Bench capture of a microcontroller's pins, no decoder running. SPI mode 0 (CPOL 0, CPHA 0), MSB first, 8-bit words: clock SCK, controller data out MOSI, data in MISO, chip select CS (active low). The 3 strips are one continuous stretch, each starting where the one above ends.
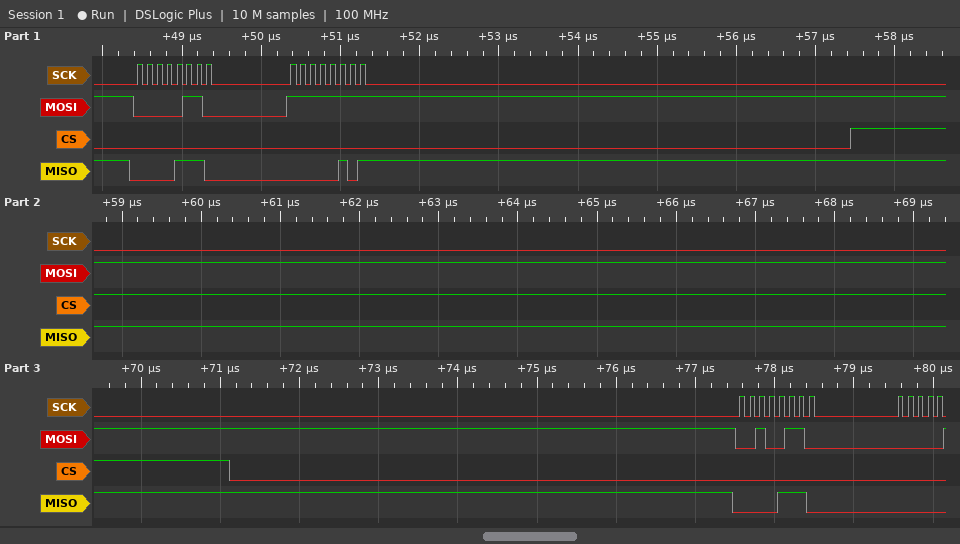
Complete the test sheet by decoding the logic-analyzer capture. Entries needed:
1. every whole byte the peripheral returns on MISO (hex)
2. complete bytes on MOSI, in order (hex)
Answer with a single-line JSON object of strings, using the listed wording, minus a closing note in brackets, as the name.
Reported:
{"every whole byte the peripheral returns on MISO": "0E 05 0E", "complete bytes on MOSI, in order": "06 FF 26"}
